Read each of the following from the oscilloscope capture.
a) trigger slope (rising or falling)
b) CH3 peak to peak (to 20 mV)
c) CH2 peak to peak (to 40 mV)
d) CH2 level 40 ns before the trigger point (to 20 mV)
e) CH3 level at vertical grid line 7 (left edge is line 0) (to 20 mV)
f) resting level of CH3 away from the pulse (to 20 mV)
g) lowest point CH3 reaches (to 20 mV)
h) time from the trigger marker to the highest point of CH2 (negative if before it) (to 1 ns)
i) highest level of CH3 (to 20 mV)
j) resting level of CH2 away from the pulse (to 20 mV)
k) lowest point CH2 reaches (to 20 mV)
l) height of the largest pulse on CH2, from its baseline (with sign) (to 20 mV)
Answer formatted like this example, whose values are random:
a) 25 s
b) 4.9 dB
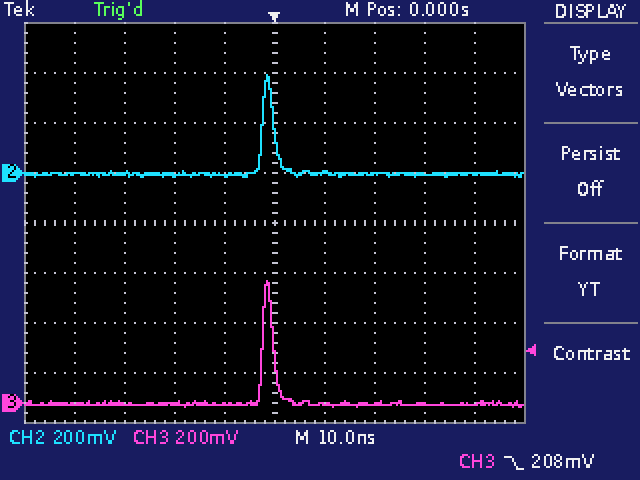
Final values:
a) falling
b) 500 mV
c) 400 mV
d) 0 mV
e) 0 mV
f) 0 mV
g) -20 mV
h) -1 ns
i) 480 mV
j) 0 mV
k) -20 mV
l) +400 mV
